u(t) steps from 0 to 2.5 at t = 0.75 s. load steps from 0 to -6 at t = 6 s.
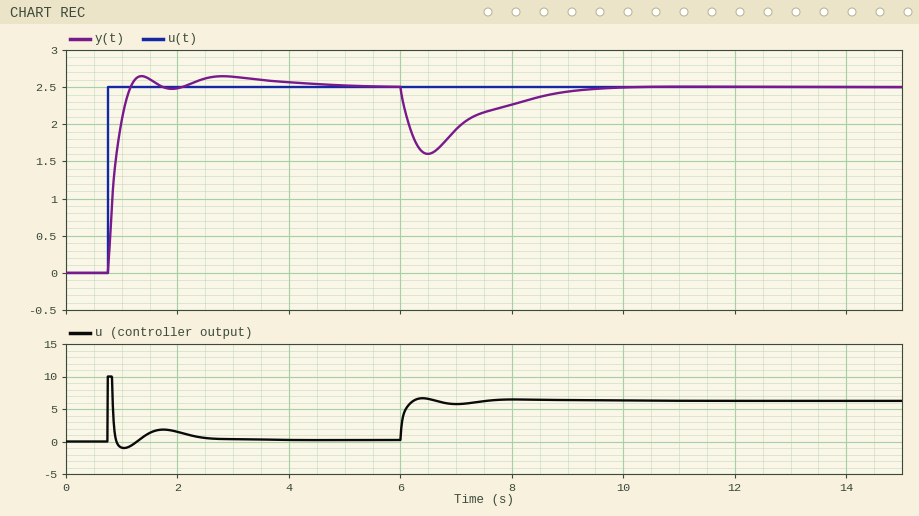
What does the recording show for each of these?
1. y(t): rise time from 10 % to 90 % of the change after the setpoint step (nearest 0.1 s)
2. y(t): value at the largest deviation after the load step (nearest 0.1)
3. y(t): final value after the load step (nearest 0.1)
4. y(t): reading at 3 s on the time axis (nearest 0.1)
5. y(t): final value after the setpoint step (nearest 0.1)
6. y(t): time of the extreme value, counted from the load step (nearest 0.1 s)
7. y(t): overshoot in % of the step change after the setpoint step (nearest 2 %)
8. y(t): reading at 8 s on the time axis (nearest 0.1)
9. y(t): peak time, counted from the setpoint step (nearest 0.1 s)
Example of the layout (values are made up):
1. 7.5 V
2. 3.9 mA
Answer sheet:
1. 0.3 s
2. 1.6
3. 2.5
4. 2.6
5. 2.5
6. 0.5 s
7. 6 %
8. 2.3
9. 0.6 s
